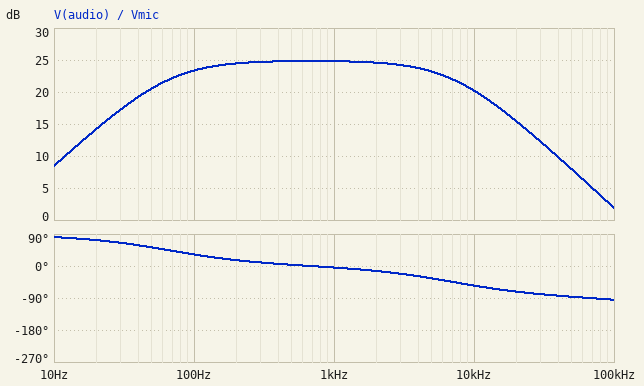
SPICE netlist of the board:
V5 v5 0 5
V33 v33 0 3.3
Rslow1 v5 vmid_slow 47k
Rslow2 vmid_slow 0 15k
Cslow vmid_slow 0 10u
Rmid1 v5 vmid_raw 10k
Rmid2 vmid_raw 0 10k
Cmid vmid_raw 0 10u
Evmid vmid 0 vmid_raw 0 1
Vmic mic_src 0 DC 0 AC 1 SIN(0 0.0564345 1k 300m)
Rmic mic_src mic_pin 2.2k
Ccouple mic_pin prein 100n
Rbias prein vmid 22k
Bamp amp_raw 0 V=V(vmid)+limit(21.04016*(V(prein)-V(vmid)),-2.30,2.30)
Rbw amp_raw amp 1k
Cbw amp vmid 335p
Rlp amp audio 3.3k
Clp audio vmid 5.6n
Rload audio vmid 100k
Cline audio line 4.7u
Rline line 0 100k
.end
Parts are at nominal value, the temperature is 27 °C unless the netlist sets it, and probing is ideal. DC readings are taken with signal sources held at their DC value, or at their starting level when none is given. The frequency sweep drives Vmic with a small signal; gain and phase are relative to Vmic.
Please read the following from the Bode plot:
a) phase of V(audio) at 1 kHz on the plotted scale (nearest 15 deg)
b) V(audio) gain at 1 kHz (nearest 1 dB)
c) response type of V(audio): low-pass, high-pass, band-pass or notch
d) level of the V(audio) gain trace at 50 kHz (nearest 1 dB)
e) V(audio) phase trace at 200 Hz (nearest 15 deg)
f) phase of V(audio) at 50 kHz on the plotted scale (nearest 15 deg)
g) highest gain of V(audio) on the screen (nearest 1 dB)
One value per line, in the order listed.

0 deg
25 dB
band-pass
8 dB
15 deg
-90 deg
25 dB
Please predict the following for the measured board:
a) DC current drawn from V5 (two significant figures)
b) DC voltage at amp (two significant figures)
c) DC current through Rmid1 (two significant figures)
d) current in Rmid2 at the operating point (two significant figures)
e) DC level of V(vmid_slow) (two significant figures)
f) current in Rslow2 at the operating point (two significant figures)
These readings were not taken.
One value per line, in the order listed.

330 µA
2.5 V
250 µA
250 µA
1.2 V
81 µA
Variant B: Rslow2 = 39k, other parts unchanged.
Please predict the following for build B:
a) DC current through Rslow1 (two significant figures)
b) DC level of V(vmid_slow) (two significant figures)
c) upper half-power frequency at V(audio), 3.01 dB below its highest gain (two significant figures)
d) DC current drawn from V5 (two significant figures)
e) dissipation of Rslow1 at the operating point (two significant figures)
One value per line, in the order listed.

58 µA
2.3 V
7.3 kHz
310 µA
160 µW
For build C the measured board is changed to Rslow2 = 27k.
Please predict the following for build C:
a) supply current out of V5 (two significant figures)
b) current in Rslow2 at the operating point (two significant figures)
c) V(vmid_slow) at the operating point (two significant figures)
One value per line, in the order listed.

320 µA
68 µA
1.8 V
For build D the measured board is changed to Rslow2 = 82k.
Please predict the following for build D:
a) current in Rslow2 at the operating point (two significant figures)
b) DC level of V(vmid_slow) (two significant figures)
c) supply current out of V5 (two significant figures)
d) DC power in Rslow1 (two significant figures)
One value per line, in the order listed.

39 µA
3.2 V
290 µA
71 µW
